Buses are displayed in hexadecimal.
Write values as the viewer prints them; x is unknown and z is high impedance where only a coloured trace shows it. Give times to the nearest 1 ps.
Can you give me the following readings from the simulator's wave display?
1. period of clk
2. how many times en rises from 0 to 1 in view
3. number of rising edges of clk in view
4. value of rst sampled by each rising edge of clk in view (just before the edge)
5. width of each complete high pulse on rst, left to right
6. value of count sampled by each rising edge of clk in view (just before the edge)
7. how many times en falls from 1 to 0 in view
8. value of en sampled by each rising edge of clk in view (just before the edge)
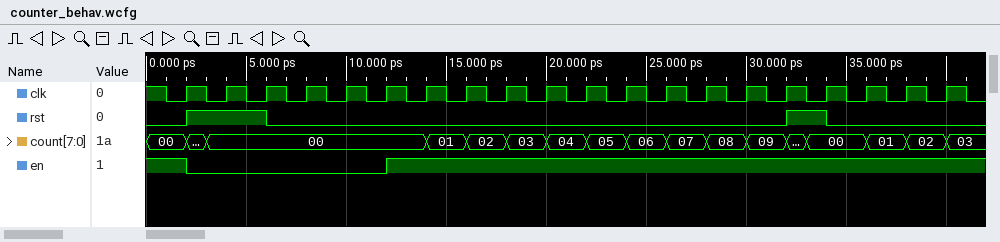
2 ps
1
20
0 1 1 0 0 0 0 0 0 0 0 0 0 0 0 0 1 0 0 0
4 ps, 2 ps
00, 00, 00, 00, 00, 00, 00, 01, 02, 03, 04, 05, 06, 07, 08, 09, 00, 00, 01, 02
1
1 0 0 0 0 0 1 1 1 1 1 1 1 1 1 1 1 1 1 1
